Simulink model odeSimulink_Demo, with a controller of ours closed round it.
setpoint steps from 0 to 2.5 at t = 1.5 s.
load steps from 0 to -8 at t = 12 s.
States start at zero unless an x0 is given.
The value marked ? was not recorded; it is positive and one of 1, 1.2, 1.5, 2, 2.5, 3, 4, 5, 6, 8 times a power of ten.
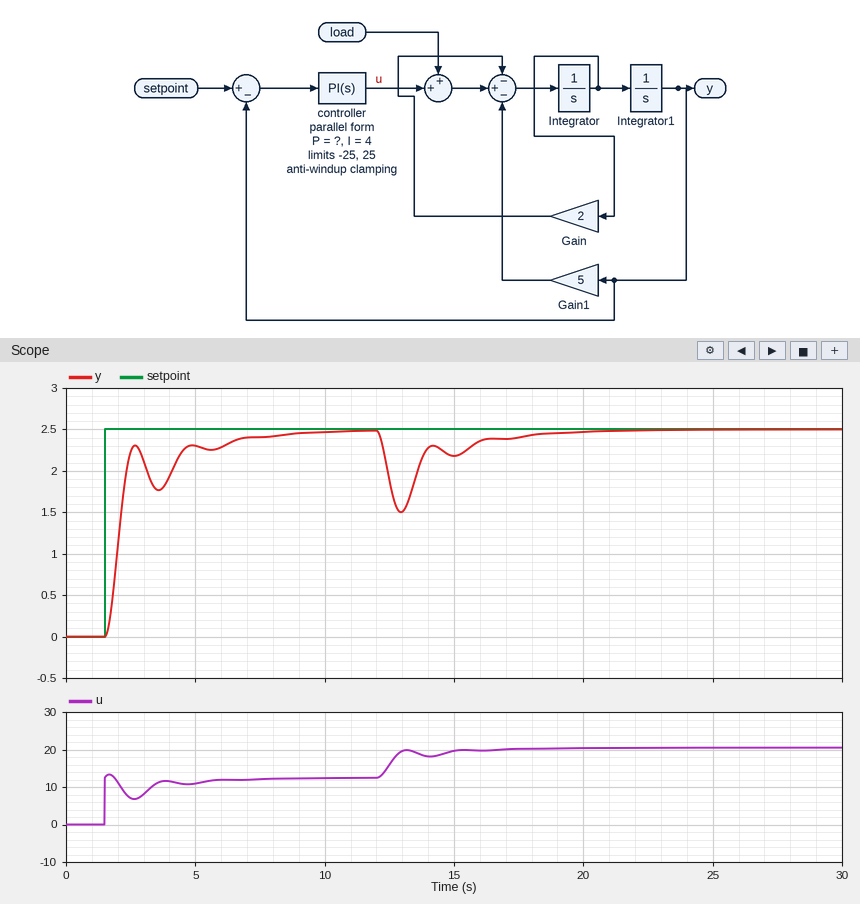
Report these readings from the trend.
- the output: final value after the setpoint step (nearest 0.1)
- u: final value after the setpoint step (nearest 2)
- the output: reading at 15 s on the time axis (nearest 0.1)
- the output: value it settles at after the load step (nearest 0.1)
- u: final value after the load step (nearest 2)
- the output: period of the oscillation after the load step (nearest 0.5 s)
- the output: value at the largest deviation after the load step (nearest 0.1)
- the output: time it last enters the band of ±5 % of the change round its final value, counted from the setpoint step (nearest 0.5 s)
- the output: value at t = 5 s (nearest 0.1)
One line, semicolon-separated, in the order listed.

2.5; 12; 2.2; 2.5; 20; 2.0 s; 1.5; 5.0 s; 2.3
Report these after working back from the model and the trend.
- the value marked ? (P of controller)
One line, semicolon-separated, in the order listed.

5
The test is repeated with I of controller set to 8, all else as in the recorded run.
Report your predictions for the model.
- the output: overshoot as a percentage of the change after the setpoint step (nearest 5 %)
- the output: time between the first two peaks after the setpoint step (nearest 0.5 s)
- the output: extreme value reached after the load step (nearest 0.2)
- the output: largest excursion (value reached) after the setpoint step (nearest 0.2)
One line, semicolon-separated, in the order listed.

15 %; 2.0 s; 1.6; 2.8
